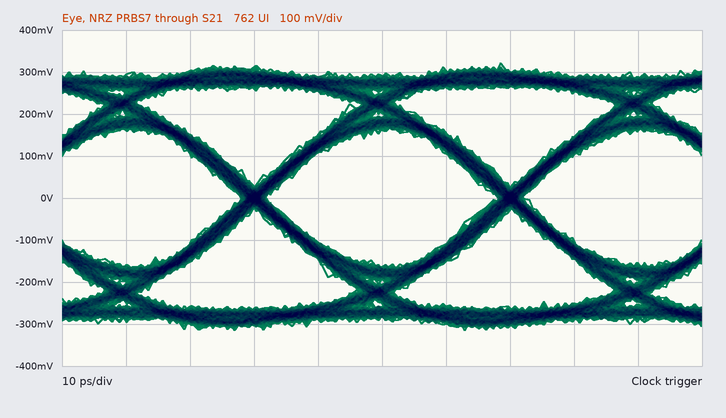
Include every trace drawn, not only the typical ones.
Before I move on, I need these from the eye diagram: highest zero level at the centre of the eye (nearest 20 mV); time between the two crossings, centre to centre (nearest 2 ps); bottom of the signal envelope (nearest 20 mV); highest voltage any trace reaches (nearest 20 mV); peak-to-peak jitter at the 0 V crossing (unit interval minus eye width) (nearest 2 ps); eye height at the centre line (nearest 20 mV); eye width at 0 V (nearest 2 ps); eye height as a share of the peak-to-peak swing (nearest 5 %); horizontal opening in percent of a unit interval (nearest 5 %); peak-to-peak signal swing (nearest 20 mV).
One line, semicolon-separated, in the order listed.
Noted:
-160 mV; 40 ps; -320 mV; 320 mV; 4 ps; 320 mV; 36 ps; 50 %; 90 %; 640 mV
